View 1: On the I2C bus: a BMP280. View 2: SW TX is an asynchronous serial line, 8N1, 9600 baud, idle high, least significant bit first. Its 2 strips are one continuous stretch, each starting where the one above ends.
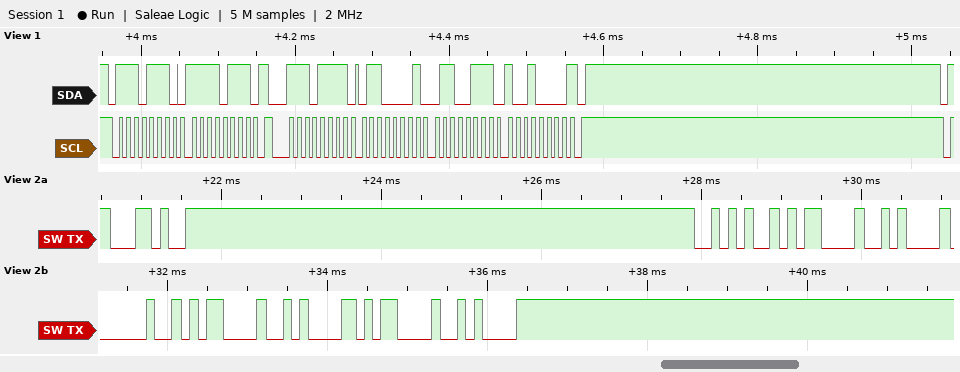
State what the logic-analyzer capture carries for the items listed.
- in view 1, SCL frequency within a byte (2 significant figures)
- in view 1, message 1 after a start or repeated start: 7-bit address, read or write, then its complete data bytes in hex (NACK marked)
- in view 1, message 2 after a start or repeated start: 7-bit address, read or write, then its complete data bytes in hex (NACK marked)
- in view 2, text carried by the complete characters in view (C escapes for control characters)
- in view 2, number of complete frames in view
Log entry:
100 kHz
0x77 write: F7
0x77 read: 61 67 90 NACK
",*\r\n \r\n\r\n"
9
